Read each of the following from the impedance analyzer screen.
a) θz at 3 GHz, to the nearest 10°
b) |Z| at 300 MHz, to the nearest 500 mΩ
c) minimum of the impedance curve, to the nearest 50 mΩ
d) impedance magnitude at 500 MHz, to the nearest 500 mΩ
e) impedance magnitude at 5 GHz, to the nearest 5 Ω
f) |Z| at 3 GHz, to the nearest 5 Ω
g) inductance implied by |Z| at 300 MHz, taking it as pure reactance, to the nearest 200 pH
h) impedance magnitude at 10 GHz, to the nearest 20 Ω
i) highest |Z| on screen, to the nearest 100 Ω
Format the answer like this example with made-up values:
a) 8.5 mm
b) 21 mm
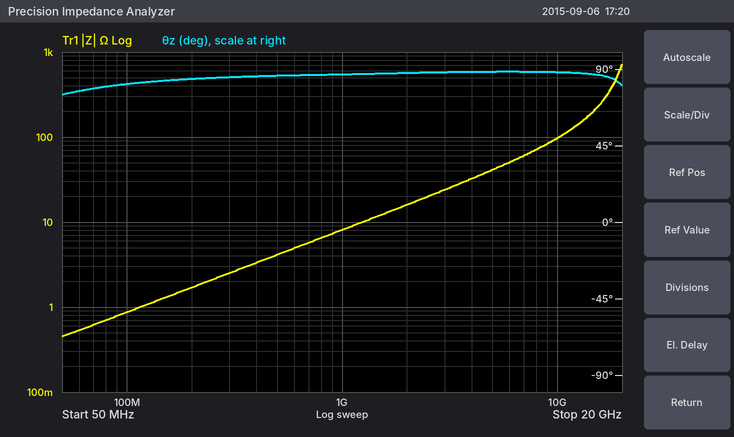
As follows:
a) 90°
b) 2.5 Ω
c) 450 mΩ
d) 4.0 Ω
e) 40 Ω
f) 25 Ω
g) 1.4 nH
h) 100 Ω
i) 700 Ω
